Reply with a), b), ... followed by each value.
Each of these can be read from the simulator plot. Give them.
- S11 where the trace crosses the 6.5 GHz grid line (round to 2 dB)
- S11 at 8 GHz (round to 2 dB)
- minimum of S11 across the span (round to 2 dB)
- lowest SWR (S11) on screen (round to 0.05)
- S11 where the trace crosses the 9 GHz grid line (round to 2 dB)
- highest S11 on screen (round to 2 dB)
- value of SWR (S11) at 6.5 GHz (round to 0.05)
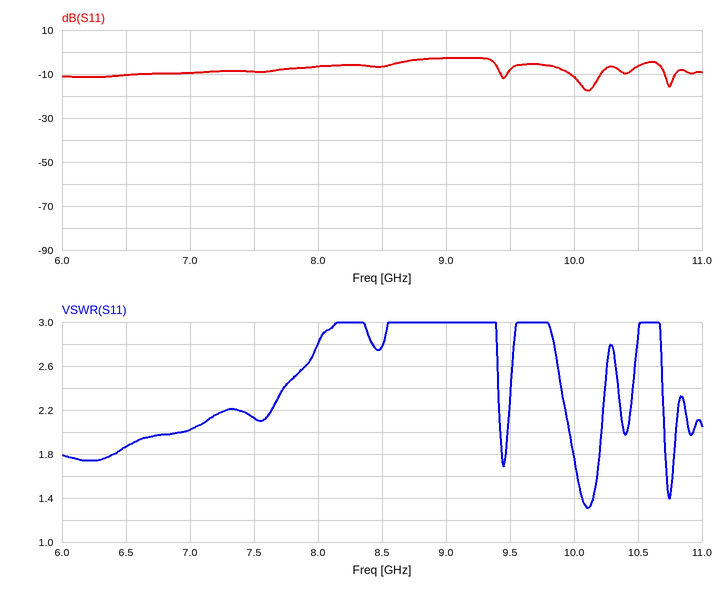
a) -10 dB
b) -6 dB
c) -18 dB
d) 1.30
e) -2 dB
f) -2 dB
g) 1.85
